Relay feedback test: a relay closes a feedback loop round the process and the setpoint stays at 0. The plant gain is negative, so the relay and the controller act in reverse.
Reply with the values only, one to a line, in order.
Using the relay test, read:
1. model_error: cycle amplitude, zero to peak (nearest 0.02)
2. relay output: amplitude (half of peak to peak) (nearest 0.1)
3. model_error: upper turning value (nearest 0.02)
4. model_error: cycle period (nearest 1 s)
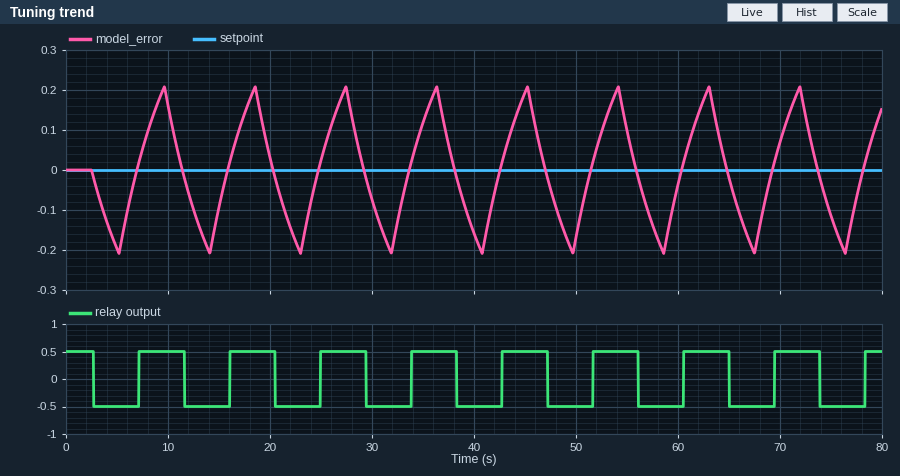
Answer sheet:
0.20
0.5
0.20
9 s
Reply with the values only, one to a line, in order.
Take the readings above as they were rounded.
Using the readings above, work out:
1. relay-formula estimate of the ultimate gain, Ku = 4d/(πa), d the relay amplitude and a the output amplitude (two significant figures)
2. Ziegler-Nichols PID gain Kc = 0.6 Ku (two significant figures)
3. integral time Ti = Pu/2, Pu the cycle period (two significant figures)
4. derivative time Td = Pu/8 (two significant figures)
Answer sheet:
3.2
1.9
4.5 s
1.1 s
